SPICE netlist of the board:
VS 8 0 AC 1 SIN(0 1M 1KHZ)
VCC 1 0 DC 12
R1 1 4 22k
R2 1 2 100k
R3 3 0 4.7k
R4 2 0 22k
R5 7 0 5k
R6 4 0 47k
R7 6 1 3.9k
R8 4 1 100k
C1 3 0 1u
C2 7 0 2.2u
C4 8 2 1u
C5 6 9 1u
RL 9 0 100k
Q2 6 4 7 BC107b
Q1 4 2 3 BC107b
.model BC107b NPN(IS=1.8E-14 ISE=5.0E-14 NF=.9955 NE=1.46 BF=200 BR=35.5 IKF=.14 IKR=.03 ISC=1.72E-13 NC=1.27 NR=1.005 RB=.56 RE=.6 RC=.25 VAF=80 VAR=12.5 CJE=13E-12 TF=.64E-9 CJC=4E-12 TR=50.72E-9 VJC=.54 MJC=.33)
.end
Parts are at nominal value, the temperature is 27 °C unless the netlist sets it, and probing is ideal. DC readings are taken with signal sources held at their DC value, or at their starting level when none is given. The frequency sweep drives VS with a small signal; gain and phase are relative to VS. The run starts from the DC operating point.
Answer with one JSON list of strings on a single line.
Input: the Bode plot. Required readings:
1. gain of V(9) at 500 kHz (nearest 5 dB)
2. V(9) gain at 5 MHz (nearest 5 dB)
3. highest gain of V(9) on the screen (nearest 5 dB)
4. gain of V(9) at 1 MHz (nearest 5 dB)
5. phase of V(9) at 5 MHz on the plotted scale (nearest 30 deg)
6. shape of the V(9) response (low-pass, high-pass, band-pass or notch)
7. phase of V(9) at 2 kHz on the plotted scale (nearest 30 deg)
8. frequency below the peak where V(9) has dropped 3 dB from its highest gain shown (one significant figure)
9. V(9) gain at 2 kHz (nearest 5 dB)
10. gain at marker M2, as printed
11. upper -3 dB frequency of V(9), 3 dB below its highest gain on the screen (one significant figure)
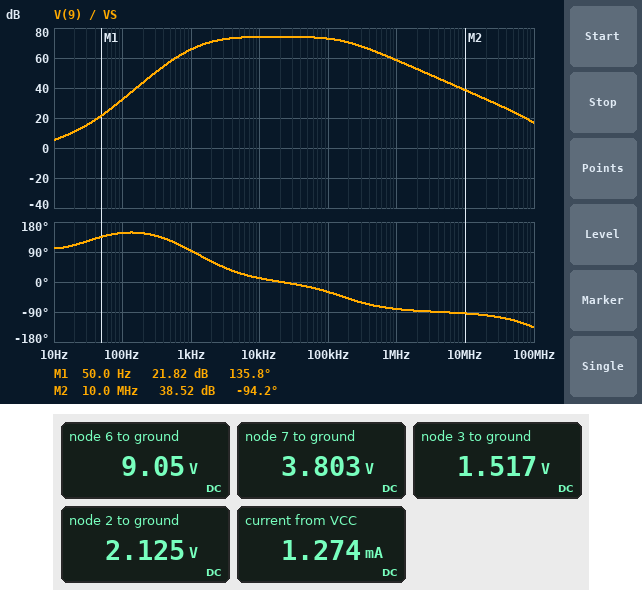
["65 dB", "45 dB", "75 dB", "60 dB", "-90 deg", "band-pass", "60 deg", "2 kHz", "70 dB", "38.52 dB", "200 kHz"]
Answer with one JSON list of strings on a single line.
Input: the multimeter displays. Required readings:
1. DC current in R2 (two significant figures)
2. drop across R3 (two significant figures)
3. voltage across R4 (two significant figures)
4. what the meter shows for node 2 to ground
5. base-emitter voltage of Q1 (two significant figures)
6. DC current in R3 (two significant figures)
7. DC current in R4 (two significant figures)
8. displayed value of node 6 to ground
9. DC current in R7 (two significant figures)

["99 µA", "1.5 V", "2.1 V", "2.125 V", "610 mV", "320 µA", "97 µA", "9.05 V", "760 µA"]
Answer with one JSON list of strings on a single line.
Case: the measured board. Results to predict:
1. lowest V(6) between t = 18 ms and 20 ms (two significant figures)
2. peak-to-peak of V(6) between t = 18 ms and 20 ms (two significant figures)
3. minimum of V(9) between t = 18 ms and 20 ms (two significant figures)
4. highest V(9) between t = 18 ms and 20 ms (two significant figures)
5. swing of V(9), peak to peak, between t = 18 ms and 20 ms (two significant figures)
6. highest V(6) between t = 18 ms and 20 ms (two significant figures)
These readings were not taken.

["7.1 V", "3.7 V", "-2.0 V", "1.8 V", "3.7 V", "11 V"]
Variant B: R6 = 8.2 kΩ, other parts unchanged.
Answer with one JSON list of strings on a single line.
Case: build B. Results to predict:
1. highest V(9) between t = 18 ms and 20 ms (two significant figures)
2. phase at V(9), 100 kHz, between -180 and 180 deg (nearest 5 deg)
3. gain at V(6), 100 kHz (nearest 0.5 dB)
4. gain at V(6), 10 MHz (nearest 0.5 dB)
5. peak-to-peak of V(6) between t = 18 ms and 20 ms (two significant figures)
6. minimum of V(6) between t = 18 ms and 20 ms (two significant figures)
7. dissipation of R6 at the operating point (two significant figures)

["620 mV", "-10 deg", "65.5 dB", "38.0 dB", "1.4 V", "10 V", "460 µW"]
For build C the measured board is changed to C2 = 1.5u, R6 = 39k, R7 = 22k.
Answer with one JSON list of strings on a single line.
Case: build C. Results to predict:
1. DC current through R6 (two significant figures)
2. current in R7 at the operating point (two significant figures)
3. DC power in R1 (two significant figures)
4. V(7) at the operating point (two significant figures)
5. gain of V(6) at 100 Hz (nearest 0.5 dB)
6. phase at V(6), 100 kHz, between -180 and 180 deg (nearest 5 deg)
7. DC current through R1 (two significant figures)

["82 µA", "430 µA", "3.5 mW", "2.6 V", "-4.0 dB", "-25 deg", "400 µA"]
